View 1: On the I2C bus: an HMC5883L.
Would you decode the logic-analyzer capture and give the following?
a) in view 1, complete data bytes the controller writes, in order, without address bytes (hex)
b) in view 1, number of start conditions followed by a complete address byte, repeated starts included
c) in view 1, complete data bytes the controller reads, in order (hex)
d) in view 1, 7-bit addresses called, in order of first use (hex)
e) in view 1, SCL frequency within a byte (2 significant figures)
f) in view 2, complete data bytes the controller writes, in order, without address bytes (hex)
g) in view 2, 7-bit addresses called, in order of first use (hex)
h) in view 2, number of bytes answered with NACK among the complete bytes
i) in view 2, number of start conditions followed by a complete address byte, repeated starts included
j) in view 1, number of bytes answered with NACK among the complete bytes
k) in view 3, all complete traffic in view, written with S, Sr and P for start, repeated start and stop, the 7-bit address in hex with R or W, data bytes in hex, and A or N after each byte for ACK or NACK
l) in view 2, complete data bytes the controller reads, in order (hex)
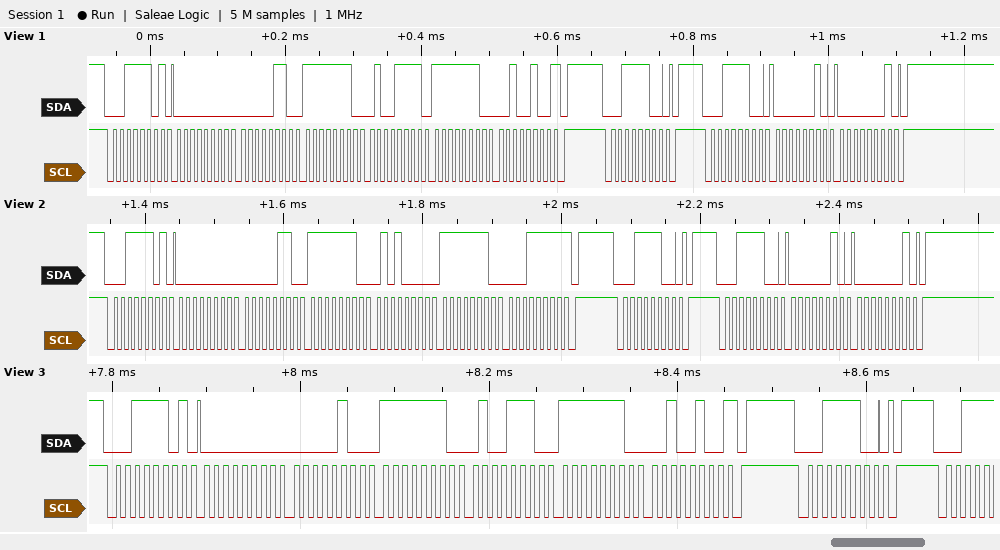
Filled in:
02 01
3
00 06 FE 4F FE 24
0x1E
100 kHz
02 01
0x1E
1
3
1
S 1ER A 00 A 04 A FE A 4E A FE A 24 N P S 1EW A P
00 06 FE 50 FE 1F
